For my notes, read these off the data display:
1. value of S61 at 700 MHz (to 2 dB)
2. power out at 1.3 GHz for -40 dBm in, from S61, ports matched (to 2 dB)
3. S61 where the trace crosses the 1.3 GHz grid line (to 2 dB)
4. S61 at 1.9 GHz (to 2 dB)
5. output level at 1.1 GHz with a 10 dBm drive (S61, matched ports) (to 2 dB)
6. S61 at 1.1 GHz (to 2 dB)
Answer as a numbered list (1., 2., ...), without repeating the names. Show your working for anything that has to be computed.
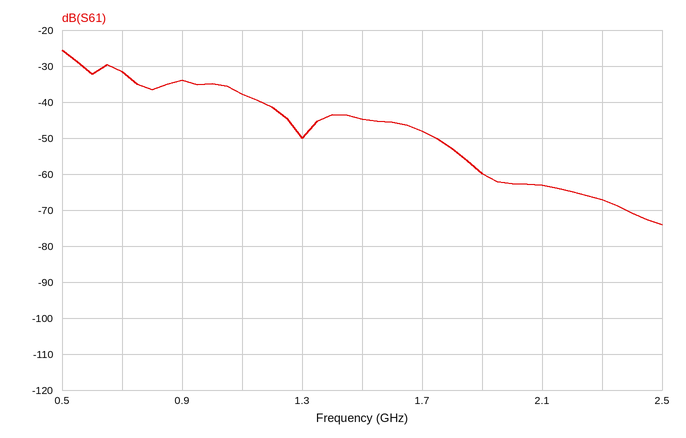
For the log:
1. -32 dB
2. -40 dBm + (-50 dB) = -90 dBm
3. -50 dB
4. -60 dB
5. 10 dBm + (-38 dB) = -28 dBm
6. -38 dB
